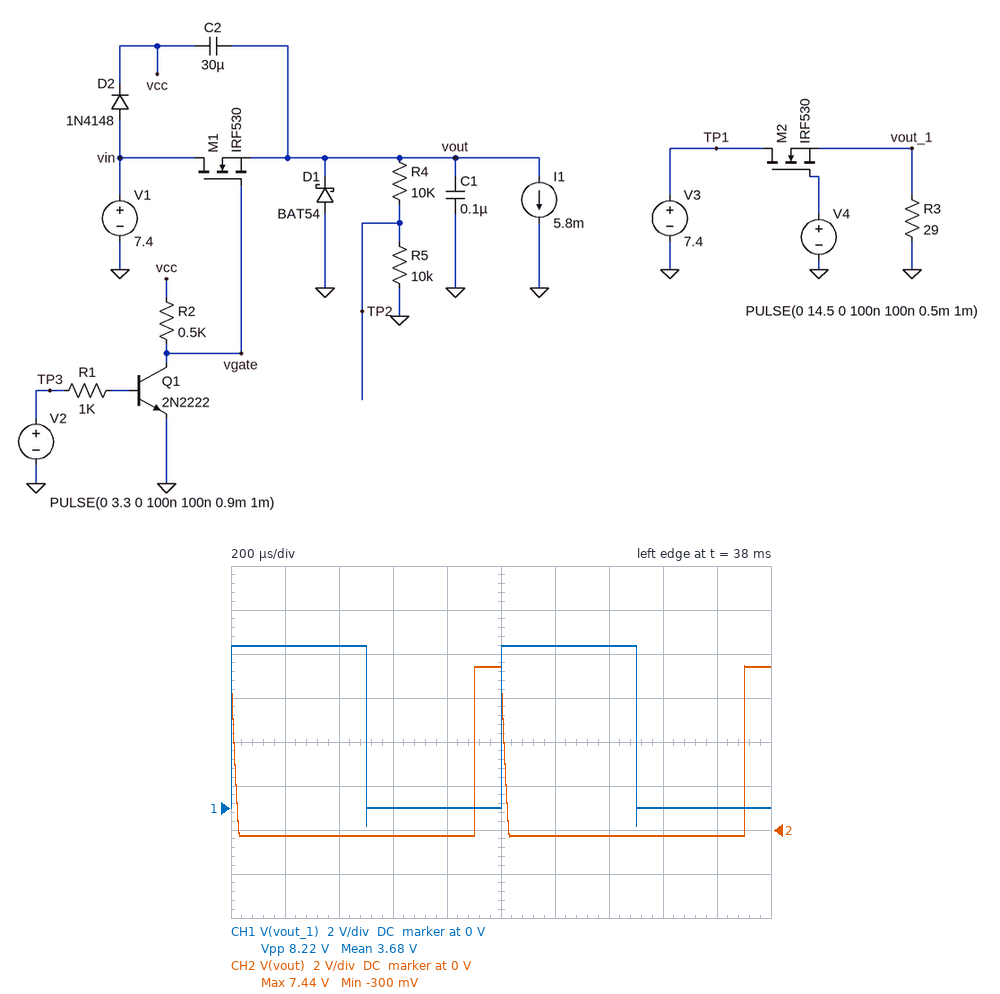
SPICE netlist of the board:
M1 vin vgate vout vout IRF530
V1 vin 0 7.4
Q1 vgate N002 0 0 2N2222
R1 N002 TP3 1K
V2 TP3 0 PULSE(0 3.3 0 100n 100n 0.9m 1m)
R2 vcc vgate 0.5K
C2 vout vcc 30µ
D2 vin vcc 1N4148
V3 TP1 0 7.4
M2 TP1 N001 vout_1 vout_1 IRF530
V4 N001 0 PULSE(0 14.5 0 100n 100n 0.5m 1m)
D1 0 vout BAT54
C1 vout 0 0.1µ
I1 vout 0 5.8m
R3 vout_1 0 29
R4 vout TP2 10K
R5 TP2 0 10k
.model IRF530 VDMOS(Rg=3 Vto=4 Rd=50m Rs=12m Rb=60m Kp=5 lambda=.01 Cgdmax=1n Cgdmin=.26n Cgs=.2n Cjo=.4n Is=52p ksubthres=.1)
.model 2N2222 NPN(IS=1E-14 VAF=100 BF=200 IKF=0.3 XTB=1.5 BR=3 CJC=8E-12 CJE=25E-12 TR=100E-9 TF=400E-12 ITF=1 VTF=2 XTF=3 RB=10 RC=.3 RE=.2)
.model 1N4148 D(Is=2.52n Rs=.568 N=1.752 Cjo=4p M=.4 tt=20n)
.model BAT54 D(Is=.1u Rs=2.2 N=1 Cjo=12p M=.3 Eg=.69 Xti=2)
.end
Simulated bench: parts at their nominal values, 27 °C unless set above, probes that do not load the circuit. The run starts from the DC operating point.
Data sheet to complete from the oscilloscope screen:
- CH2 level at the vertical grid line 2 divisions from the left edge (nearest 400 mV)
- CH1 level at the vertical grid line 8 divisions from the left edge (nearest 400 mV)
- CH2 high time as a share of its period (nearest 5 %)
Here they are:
-400 mV
0 V
10 %
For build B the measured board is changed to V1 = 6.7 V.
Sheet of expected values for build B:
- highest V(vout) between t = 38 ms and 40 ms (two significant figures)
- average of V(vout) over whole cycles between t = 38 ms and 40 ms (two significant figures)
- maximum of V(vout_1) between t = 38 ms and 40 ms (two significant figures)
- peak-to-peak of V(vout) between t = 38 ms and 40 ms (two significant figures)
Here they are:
6.7 V
490 mV
7.4 V
7.0 V
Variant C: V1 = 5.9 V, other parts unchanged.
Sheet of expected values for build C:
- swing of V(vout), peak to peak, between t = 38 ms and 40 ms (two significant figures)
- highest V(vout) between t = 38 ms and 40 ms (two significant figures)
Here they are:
6.2 V
5.9 V
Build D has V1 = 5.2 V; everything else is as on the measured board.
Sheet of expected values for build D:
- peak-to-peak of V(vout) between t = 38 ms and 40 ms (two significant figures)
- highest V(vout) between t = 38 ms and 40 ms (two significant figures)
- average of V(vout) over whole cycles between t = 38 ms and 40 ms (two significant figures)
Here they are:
5.5 V
5.2 V
310 mV
